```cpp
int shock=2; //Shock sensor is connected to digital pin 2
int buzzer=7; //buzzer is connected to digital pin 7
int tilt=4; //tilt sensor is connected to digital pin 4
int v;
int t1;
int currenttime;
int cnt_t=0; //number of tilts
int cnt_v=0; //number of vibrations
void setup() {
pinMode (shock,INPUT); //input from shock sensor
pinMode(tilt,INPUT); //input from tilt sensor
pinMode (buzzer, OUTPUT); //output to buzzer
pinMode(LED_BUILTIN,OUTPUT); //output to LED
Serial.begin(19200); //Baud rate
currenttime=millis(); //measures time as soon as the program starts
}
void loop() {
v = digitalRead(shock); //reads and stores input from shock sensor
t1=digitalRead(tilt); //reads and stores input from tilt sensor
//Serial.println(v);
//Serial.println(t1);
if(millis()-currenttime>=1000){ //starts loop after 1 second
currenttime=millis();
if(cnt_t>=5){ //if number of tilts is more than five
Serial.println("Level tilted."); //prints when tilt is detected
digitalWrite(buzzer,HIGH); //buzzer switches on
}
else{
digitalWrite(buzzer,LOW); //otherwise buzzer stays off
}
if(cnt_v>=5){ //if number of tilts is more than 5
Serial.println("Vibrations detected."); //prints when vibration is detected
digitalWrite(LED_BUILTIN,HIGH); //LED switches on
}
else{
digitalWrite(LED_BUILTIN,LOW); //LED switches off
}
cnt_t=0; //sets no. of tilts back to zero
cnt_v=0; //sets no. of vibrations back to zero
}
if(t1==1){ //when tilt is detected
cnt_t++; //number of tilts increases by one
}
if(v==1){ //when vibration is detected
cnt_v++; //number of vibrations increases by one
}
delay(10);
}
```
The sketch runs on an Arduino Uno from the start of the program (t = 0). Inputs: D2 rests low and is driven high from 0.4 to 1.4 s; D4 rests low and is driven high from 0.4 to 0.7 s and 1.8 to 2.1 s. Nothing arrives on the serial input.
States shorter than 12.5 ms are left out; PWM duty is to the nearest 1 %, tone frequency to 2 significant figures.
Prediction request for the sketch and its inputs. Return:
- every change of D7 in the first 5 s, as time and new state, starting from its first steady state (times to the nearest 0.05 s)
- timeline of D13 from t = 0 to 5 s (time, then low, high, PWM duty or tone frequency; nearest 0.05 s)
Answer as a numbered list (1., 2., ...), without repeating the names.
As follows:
1. 0 s low; 1 s high; 4 s low
2. 0 s low; 1 s high; 3 s low
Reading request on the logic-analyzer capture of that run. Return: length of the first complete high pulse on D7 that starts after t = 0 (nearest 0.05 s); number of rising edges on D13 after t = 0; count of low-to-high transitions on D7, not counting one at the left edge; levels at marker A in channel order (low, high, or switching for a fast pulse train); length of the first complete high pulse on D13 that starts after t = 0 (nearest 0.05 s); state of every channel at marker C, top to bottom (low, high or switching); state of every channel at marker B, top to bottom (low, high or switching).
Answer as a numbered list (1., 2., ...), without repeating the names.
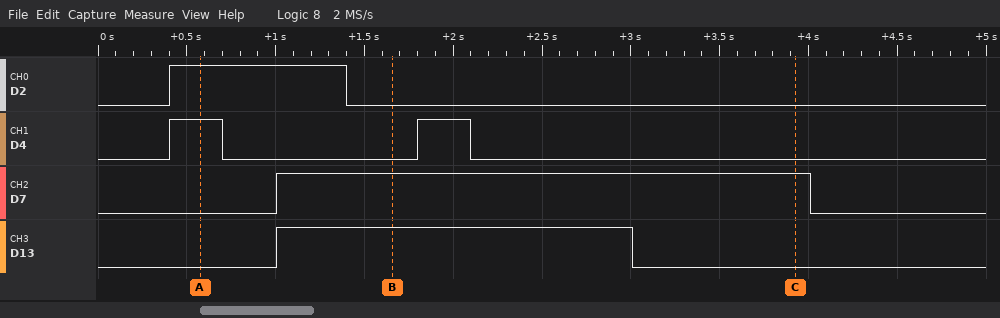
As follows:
1. 3.00 s
2. 1
3. 1
4. D2 high, D4 high, D7 low, D13 low
5. 2.00 s
6. D2 low, D4 low, D7 high, D13 low
7. D2 low, D4 low, D7 high, D13 high
